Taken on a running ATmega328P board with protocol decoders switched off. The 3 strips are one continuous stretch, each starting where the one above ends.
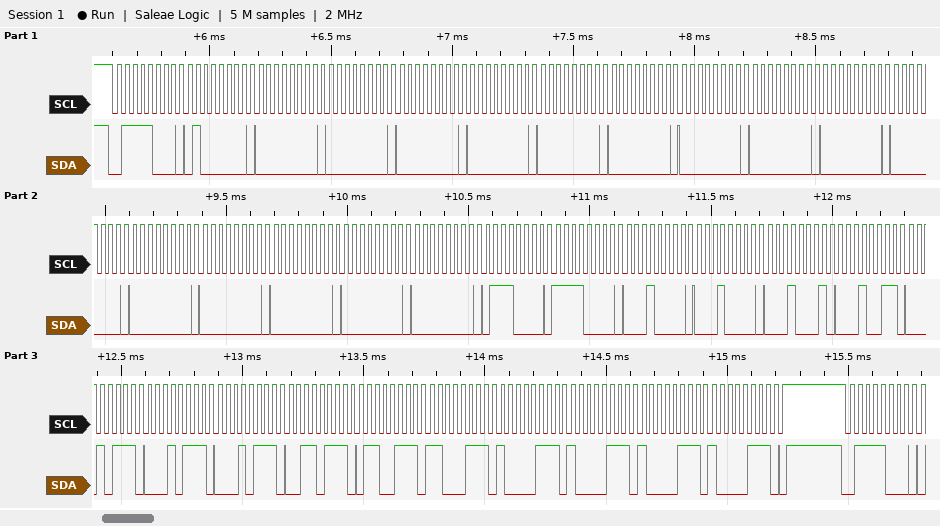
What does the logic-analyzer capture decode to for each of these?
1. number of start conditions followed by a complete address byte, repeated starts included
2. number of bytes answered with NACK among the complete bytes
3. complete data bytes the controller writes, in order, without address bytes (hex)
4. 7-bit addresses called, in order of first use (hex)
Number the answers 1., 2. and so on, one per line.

1. 2
2. 0
3. 40 00 00 00 00 00 00 00 00 00 00 00 00 00 00 00 70 F0 10 10 11 13 17 17 17 37 67 C7 87 87 87 87
4. 0x3C
